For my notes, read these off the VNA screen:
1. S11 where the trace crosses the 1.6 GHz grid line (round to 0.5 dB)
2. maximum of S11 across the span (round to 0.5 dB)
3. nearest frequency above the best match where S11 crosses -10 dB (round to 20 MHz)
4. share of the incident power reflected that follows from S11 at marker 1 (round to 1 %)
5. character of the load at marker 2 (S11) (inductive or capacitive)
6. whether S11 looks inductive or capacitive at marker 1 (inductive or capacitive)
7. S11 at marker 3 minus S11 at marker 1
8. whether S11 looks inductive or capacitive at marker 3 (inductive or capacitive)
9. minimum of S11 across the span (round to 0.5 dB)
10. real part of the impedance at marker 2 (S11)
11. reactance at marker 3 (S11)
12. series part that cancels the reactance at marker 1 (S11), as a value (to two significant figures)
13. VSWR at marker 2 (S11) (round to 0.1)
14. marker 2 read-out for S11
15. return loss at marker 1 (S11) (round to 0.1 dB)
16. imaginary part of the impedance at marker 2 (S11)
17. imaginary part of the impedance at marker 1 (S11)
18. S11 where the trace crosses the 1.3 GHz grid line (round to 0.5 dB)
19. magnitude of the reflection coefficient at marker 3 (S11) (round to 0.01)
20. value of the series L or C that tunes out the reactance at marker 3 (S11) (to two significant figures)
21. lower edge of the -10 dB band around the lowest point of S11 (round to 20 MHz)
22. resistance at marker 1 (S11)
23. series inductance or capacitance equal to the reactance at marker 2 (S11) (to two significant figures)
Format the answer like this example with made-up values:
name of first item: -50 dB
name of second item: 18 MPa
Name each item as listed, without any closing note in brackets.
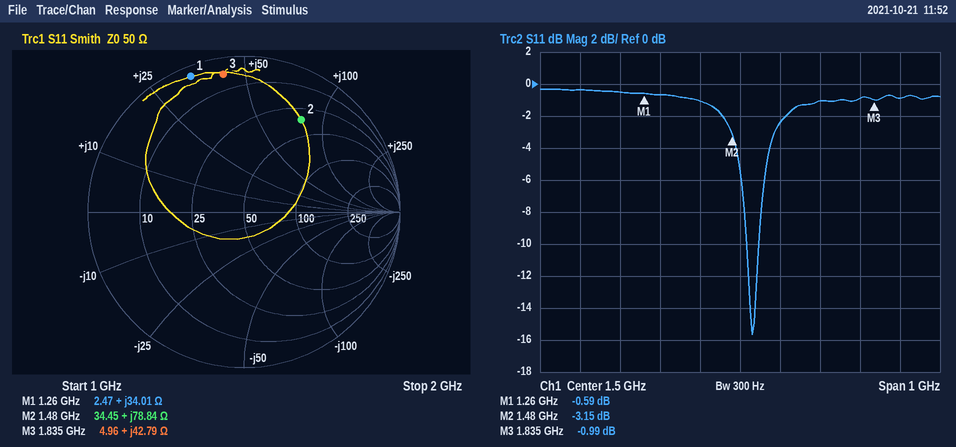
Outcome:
S11 where the trace crosses the 1.6 GHz grid line: -2.5 dB
maximum of S11 across the span: -0.5 dB
nearest frequency above the best match where S11 crosses -10 dB: 1.54 GHz
share of the incident power reflected that follows from S11 at marker 1: 87 %
character of the load at marker 2 (S11): inductive
whether S11 looks inductive or capacitive at marker 1: inductive
S11 at marker 3 minus S11 at marker 1: -0.40 dB
whether S11 looks inductive or capacitive at marker 3: inductive
minimum of S11 across the span: -15.5 dB
real part of the impedance at marker 2: 34.45 Ω
reactance at marker 3: +42.79 Ω
series part that cancels the reactance at marker 1 (S11), as a value: 3.7 pF
VSWR at marker 2 (S11): 5.6
marker 2 read-out for S11: -3.15 dB
return loss at marker 1 (S11): 0.6 dB
imaginary part of the impedance at marker 2: +78.84 Ω
imaginary part of the impedance at marker 1: +34.01 Ω
S11 where the trace crosses the 1.3 GHz grid line: -0.5 dB
magnitude of the reflection coefficient at marker 3 (S11): 0.89
value of the series L or C that tunes out the reactance at marker 3 (S11): 2.0 pF
lower edge of the -10 dB band around the lowest point of S11: 1.52 GHz
resistance at marker 1: 2.47 Ω
series inductance or capacitance equal to the reactance at marker 2 (S11): 8.5 nH
